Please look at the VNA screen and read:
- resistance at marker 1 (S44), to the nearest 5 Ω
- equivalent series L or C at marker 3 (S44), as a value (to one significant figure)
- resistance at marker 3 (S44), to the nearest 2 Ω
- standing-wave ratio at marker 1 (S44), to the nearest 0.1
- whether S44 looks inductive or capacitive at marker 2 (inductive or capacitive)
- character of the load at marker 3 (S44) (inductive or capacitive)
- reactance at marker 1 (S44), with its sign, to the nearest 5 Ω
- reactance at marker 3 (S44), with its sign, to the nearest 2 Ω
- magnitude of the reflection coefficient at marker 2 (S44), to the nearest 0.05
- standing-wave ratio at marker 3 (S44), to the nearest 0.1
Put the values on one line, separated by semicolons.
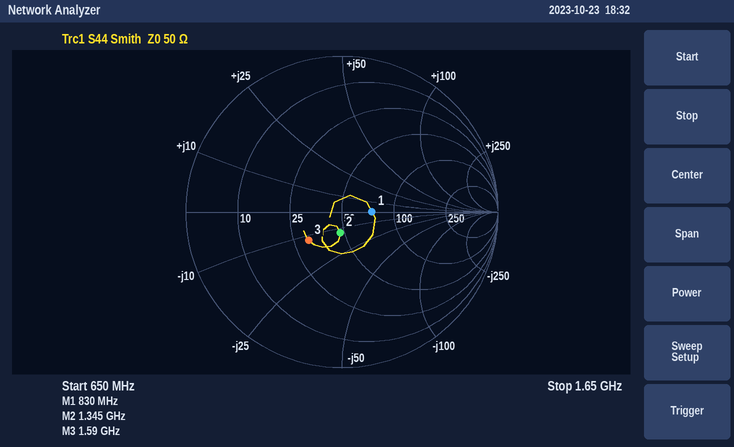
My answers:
75 Ω; 8 pF; 30 Ω; 1.5; capacitive; capacitive; 0 Ω; -12 Ω; 0.15; 1.8
